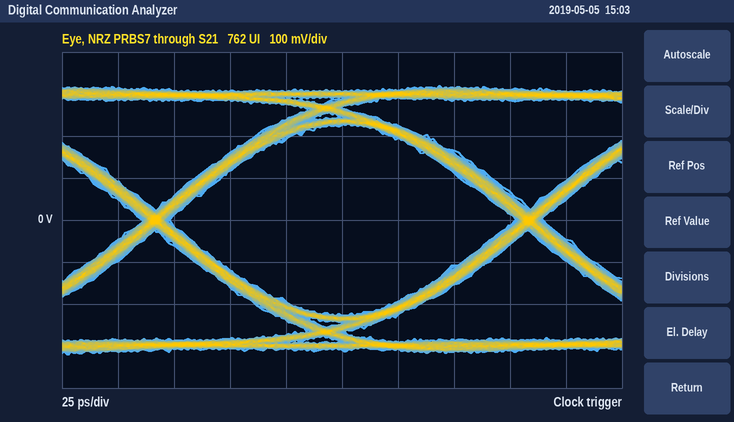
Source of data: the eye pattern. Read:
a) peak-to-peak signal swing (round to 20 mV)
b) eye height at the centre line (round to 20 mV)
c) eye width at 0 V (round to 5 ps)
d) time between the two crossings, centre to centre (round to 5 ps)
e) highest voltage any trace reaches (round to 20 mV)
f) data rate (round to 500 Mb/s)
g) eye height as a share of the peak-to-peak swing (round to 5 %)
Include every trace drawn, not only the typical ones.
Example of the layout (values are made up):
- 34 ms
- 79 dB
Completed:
- 640 mV
- 460 mV
- 155 ps
- 165 ps
- 320 mV
- 6.0 Gb/s
- 70 %
